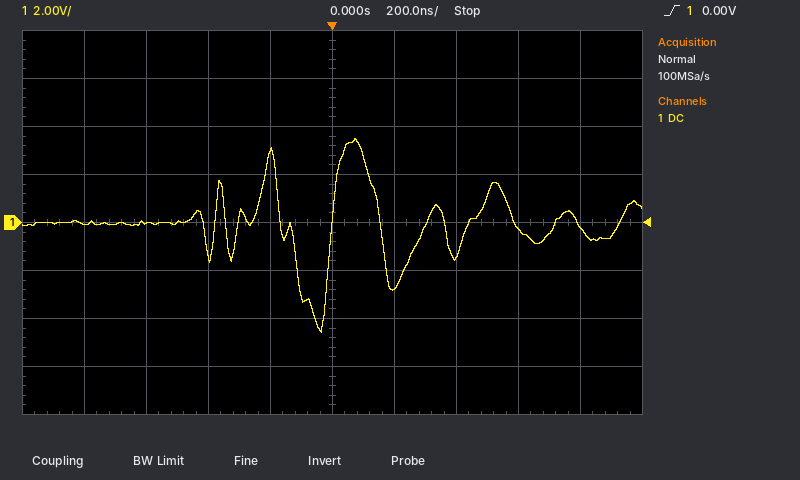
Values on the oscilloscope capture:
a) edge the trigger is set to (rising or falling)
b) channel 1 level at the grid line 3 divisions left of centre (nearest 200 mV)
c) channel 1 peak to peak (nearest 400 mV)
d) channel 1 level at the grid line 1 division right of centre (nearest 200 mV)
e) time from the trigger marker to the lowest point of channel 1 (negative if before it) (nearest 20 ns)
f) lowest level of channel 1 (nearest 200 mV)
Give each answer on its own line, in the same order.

rising
0.0 V
8.0 V
-2.8 V
-40 ns
-4.6 V
